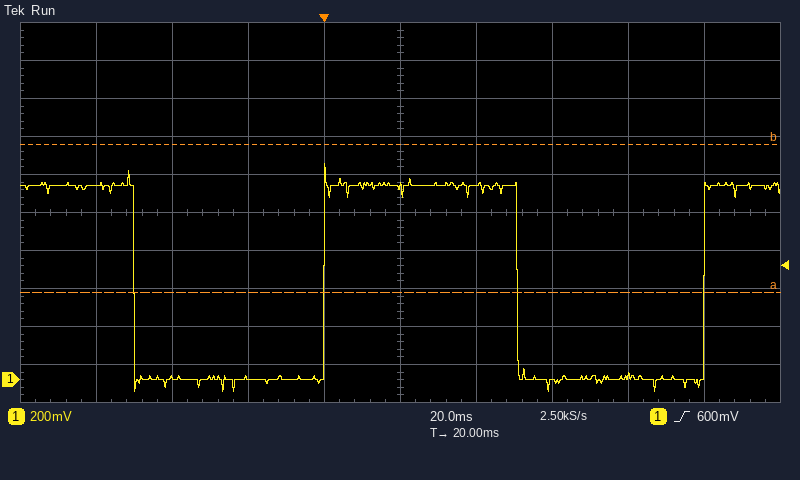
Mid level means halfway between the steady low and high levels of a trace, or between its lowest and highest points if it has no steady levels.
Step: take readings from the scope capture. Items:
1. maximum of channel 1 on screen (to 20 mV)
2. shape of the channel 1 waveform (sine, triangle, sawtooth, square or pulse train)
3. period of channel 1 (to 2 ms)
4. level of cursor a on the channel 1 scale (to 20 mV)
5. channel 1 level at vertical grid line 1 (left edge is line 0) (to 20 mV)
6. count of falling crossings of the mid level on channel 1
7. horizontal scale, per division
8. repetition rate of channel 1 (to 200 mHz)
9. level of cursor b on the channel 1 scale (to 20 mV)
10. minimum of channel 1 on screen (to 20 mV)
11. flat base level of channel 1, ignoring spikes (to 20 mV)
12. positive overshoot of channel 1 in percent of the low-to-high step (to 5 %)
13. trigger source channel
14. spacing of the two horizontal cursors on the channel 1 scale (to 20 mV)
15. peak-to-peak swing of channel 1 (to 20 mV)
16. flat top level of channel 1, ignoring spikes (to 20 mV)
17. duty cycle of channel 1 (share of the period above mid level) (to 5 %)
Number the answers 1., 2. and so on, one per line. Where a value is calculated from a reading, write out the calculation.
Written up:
1. 1.14 V
2. square
3. 100 ms
4. 460 mV
5. 1.02 V
6. 2
7. 20 ms
8. 1 / 100 ms ≈ 10.0 Hz
9. 1.24 V
10. -60 mV
11. 0 mV
12. 10 %
13. channel 1
14. 780 mV
15. 1.14 V − (-60 mV) = 1.20 V
16. 1.02 V
17. 50 %
